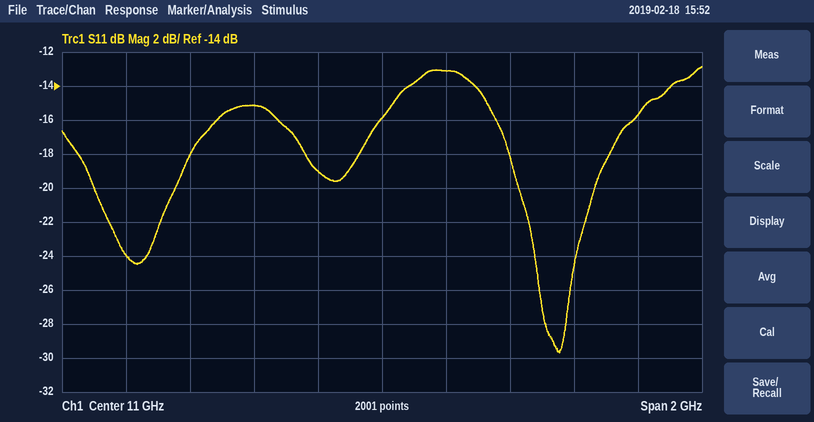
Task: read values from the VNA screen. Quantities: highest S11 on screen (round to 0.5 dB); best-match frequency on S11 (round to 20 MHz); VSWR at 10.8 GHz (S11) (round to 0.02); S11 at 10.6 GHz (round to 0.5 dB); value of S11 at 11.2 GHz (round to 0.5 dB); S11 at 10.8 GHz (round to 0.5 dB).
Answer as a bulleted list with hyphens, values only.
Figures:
- -13.0 dB
- 11.56 GHz
- 1.26
- -15.0 dB
- -13.0 dB
- -19.0 dB
